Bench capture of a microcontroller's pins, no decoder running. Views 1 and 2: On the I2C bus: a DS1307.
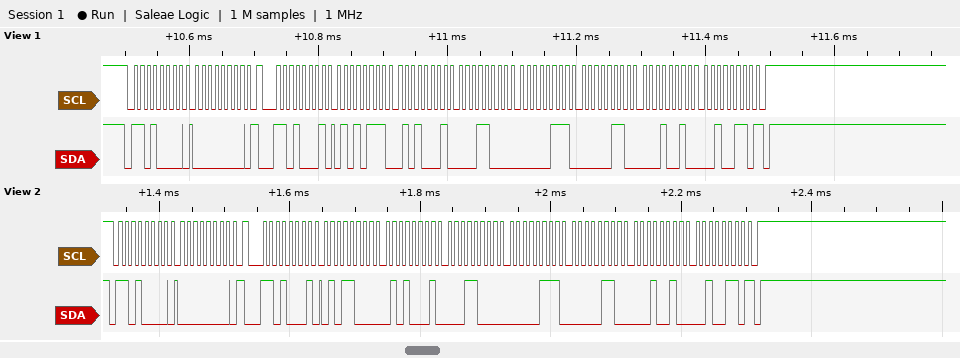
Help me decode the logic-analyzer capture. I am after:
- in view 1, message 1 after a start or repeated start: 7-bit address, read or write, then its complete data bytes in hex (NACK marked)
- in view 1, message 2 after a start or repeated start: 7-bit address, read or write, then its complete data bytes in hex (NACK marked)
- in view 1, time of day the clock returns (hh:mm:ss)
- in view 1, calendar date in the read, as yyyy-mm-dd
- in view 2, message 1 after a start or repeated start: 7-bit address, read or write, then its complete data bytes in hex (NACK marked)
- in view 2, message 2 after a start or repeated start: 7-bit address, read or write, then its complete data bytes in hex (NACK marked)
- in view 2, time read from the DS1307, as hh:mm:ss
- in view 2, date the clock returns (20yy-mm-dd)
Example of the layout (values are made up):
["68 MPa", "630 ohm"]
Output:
["0x68 write: 00", "0x68 read: 57 51 18 07 06 12 26 NACK", "18:51:57", "2026-12-06", "0x68 write: 00", "0x68 read: 58 51 18 07 06 12 26 NACK", "18:51:58", "2026-12-06"]
